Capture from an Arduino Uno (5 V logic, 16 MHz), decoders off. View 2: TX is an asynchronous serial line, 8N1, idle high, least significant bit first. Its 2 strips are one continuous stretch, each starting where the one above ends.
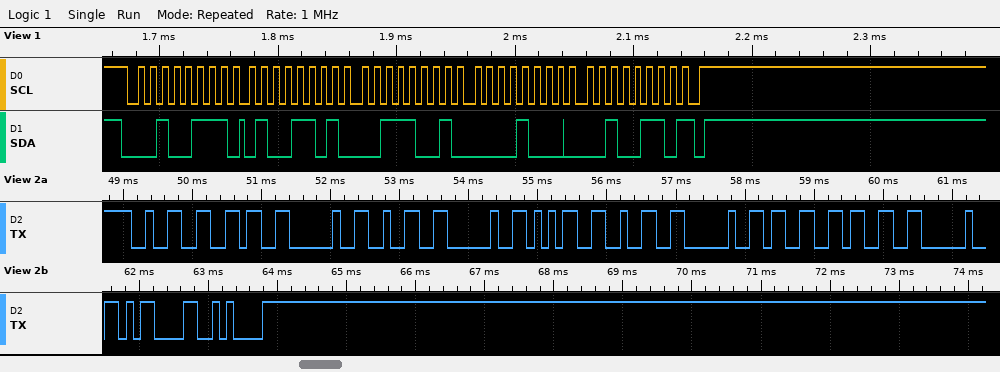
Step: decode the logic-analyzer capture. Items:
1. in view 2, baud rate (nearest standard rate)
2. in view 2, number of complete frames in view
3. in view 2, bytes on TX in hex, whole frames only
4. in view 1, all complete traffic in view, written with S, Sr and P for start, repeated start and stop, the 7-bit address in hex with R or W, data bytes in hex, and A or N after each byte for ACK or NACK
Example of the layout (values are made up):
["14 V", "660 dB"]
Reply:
["9600 baud", "13", "0x32 0x36 0x20 0x32 0x20 0x35 0x32 0x20 0x33 0x33 0x20 0x0D 0x0A", "S 13R A 4D A 39 A 08 A 26 N P"]
